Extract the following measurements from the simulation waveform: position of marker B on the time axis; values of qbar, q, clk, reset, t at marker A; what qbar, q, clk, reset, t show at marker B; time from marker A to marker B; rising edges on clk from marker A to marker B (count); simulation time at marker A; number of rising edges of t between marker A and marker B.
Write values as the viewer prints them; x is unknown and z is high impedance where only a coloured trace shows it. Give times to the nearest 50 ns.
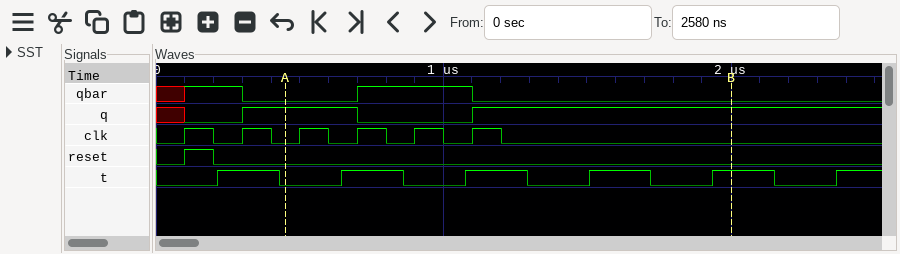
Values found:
2000 ns
qbar=0, q=1, clk=0, reset=0, t=0
qbar=0, q=1, clk=0, reset=0, t=1
1550 ns
4
450 ns
4
